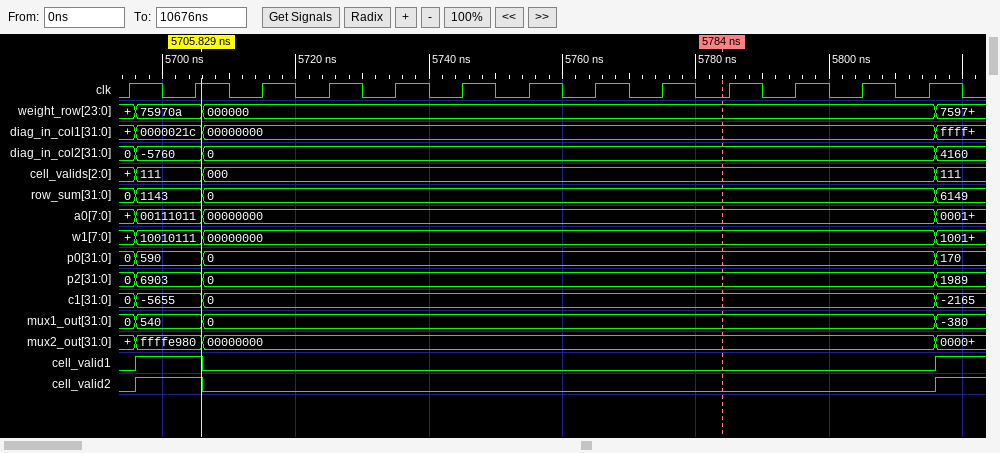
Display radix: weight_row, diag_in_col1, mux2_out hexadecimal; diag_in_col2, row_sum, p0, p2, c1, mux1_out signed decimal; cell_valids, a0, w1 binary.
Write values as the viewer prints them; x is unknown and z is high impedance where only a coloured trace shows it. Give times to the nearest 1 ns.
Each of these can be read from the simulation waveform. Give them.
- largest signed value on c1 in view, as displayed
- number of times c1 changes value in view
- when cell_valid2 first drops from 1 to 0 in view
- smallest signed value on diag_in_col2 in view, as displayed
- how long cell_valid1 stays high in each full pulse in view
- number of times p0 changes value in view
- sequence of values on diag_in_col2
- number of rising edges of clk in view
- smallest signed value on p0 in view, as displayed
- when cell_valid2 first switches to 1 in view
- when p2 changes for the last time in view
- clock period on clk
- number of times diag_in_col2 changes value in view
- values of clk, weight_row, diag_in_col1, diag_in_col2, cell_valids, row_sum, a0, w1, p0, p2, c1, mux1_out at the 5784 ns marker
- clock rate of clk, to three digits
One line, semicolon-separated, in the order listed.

0; 3; 5706 ns; -5760; 10 ns; 3; 0, -5760, 0, 4160; 13; 0; 5696 ns; 5816 ns; 10 ns; 3; clk=0, weight_row=000000, diag_in_col1=00000000, diag_in_col2=0, cell_valids=000, row_sum=0, a0=00000000, w1=00000000, p0=0, p2=0, c1=0, mux1_out=0; 100 MHz
